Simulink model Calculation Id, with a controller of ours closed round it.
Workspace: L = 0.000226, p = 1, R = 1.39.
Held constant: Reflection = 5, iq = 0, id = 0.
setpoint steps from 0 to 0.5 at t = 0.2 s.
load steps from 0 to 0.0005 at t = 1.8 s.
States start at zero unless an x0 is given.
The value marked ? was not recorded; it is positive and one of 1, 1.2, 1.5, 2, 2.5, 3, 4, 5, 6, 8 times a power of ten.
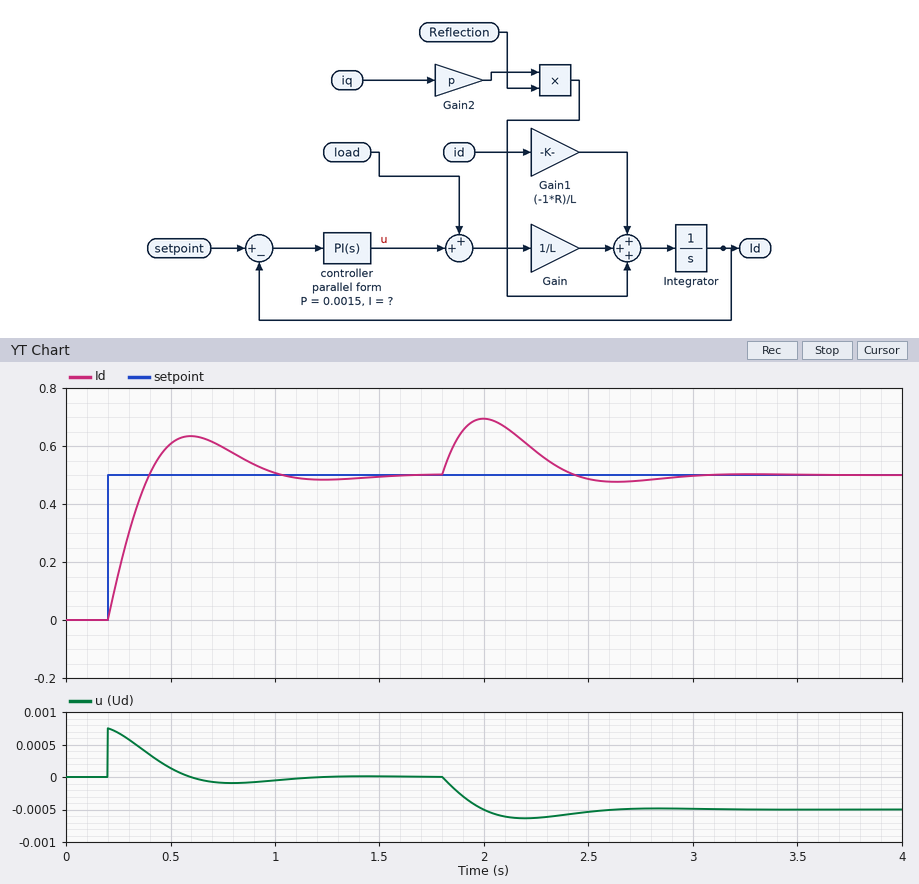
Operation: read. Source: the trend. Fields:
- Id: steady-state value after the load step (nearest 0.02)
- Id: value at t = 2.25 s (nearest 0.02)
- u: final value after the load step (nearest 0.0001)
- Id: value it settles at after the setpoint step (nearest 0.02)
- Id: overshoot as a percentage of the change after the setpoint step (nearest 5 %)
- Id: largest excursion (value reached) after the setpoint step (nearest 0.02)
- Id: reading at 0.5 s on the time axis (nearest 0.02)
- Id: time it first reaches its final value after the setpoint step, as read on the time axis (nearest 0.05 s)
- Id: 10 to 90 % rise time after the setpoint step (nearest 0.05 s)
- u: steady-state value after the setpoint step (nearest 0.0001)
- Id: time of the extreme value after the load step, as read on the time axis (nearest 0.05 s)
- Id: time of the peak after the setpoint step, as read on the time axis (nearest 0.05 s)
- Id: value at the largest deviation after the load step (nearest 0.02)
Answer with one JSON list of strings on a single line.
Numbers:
["0.50", "0.58", "-0.0005", "0.50", "25 %", "0.64", "0.60", "0.40 s", "0.15 s", "0.0000", "2.00 s", "0.60 s", "0.70"]
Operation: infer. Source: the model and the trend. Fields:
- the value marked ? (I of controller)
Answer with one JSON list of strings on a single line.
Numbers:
["0.008"]
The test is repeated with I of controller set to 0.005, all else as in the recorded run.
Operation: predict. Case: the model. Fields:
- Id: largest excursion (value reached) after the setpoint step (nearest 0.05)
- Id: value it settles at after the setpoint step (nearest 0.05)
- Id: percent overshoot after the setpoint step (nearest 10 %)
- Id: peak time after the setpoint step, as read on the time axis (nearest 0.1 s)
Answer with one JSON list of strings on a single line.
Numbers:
["0.60", "0.50", "20 %", "0.7 s"]
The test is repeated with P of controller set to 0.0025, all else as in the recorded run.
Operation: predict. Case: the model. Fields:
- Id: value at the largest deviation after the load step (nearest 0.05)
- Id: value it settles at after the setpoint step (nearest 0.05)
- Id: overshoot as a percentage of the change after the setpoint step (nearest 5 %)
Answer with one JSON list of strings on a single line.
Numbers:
["0.65", "0.50", "15 %"]
